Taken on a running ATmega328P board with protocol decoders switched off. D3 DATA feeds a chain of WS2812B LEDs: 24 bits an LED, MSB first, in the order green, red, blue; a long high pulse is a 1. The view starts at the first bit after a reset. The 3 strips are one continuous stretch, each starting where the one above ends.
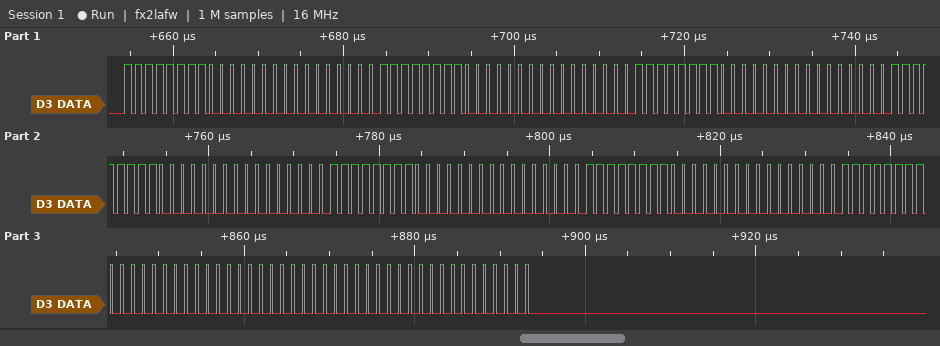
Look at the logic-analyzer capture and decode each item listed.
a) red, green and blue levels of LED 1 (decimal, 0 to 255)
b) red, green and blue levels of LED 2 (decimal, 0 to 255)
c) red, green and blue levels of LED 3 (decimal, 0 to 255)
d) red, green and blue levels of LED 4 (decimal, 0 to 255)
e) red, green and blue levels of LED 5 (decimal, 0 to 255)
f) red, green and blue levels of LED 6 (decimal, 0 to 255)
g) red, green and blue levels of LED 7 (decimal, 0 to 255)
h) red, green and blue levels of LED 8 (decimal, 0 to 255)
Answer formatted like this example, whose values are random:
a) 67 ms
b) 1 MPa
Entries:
a) 0, 255, 0
b) 0, 255, 0
c) 0, 255, 0
d) 0, 255, 0
e) 0, 255, 0
f) 0, 255, 0
g) 0, 255, 0
h) 0, 0, 0
